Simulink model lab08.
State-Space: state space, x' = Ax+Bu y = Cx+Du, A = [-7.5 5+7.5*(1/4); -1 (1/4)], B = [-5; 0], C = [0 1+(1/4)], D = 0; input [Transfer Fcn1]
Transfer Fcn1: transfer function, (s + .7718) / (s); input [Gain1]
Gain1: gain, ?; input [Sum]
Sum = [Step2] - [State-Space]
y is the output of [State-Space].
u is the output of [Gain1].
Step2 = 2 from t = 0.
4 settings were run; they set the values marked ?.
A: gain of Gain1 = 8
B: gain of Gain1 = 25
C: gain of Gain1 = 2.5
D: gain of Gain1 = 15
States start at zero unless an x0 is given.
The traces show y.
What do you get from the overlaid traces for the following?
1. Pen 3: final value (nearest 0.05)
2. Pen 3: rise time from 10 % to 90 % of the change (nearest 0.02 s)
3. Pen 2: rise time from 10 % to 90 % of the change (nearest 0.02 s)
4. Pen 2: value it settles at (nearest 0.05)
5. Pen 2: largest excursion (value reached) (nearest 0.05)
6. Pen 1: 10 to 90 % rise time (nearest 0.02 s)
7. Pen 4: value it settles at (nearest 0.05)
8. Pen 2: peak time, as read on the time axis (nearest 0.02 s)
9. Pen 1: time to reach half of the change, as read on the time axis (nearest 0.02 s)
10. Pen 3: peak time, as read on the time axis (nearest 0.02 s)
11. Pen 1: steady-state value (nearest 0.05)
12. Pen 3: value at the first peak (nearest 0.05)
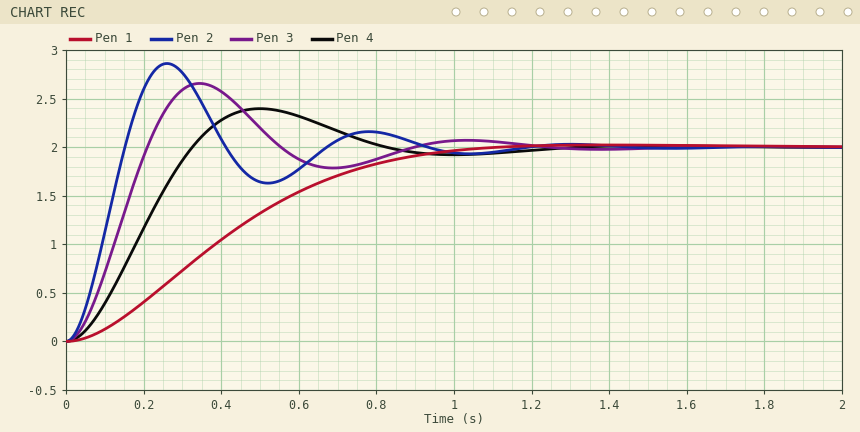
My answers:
2.00
0.14 s
0.10 s
2.00
2.85
0.64 s
2.00
0.26 s
0.38 s
0.34 s
2.00
2.65
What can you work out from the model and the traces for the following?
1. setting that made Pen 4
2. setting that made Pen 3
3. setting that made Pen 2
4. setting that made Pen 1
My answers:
A
D
B
C
